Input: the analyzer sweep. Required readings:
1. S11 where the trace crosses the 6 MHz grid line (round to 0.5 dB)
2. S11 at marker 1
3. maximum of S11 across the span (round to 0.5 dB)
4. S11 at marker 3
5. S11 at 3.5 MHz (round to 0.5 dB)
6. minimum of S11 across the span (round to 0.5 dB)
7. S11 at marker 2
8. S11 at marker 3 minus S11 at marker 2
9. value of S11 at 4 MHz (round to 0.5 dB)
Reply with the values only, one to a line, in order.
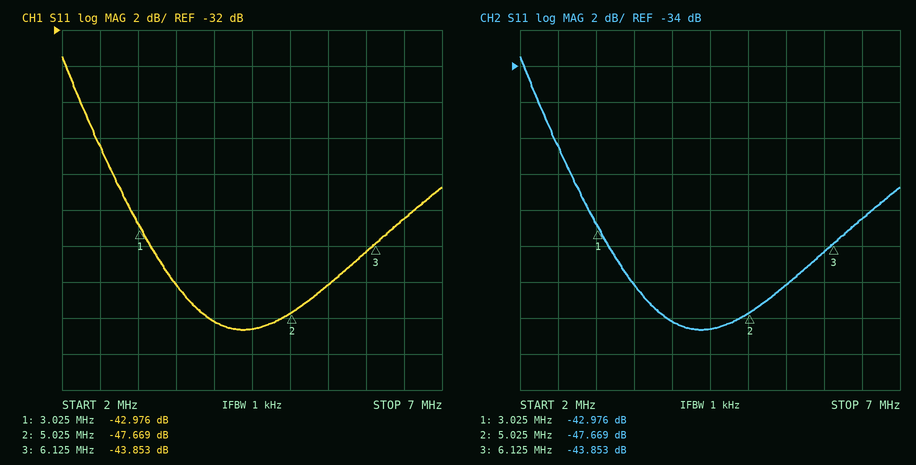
-44.5 dB
-42.976 dB
-33.5 dB
-43.853 dB
-46.0 dB
-48.5 dB
-47.669 dB
3.816 dB
-48.0 dB
